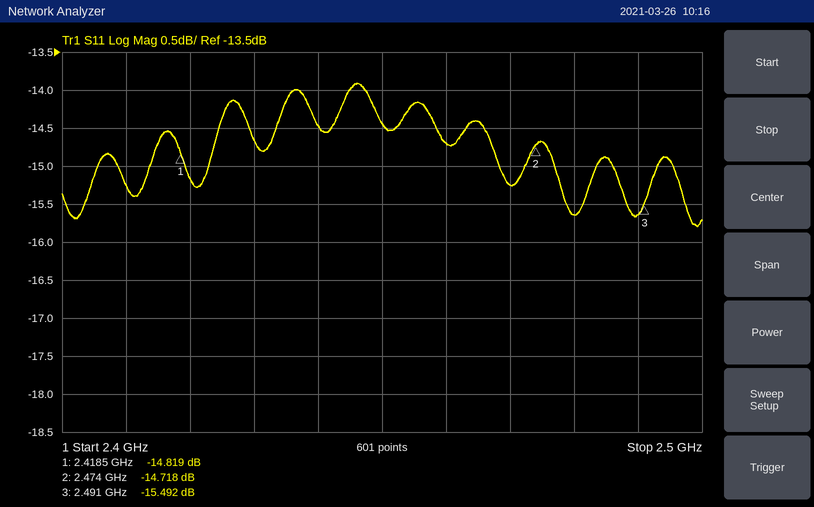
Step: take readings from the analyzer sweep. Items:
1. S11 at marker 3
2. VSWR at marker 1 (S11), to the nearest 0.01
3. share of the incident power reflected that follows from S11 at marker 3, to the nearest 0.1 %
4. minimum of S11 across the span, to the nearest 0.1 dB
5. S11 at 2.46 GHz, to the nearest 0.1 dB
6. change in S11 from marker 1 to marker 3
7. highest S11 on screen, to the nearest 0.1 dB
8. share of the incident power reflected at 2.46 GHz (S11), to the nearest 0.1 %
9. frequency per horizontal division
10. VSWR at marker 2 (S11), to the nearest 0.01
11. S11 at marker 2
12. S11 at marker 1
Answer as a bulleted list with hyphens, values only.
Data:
- -15.492 dB
- 1.44
- 2.8 %
- -15.8 dB
- -14.7 dB
- -0.673 dB
- -13.9 dB
- 3.4 %
- 10 MHz
- 1.45
- -14.718 dB
- -14.819 dB
